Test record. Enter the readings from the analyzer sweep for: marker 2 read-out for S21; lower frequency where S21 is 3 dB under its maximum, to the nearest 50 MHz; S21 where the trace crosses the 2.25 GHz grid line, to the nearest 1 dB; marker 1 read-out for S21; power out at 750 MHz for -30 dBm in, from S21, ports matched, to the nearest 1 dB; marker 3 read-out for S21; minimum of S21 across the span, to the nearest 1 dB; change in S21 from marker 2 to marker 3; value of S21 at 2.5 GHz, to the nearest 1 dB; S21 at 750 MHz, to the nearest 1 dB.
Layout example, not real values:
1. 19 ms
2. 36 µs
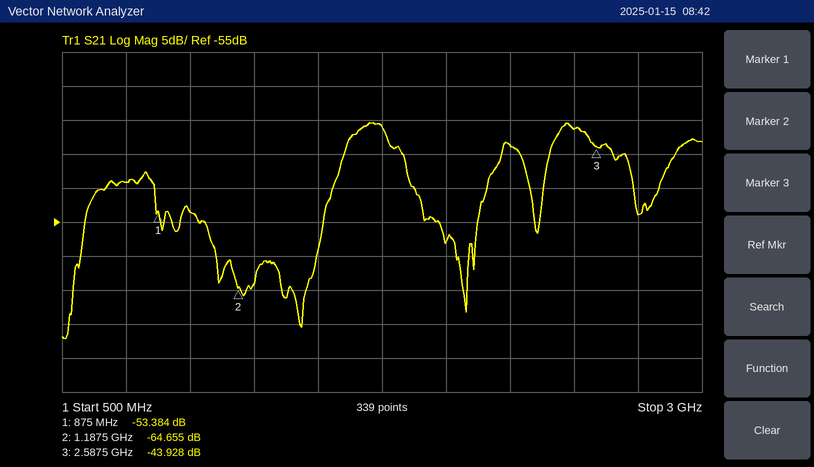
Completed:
1. -64.655 dB
2. 1.60 GHz
3. -44 dB
4. -53.384 dB
5. -79 dBm
6. -43.928 dB
7. -72 dB
8. 20.727 dB
9. -41 dB
10. -49 dB
